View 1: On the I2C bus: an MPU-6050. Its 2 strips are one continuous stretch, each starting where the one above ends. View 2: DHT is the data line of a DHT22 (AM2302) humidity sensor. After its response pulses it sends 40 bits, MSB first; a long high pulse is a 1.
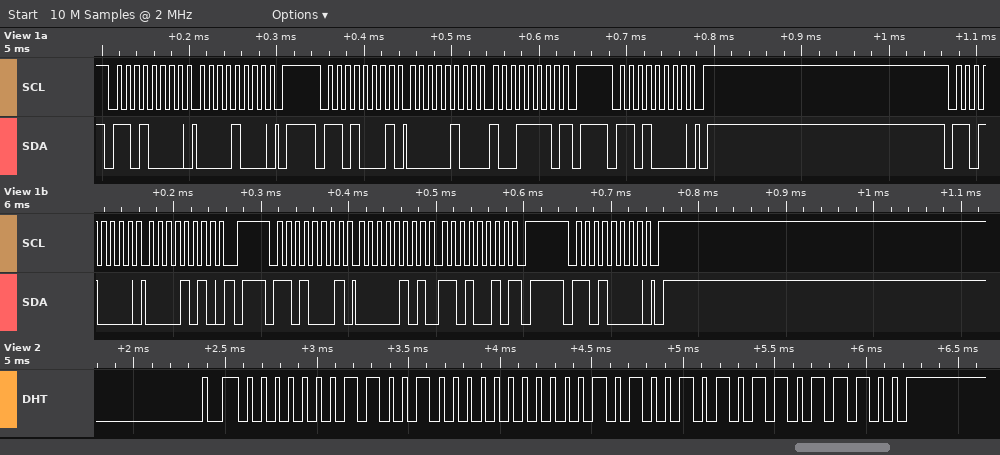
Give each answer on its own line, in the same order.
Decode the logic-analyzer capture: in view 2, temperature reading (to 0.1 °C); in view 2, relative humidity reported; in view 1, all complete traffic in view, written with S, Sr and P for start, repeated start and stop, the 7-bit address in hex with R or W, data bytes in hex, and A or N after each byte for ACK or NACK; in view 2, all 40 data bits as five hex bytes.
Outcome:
33.0 °C
40.0 %
S 68W A 08 A P S 68R A 04 A 9E N P S 68W A P S 68W A 0A A P S 68R A 05 A D2 N P S 68W A P
01 90 01 4A DC
